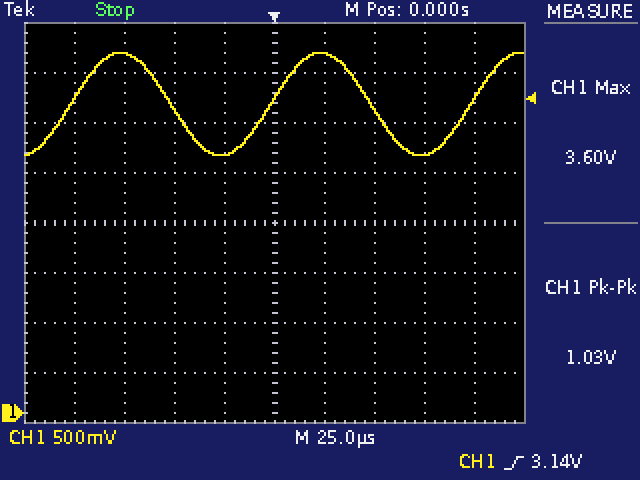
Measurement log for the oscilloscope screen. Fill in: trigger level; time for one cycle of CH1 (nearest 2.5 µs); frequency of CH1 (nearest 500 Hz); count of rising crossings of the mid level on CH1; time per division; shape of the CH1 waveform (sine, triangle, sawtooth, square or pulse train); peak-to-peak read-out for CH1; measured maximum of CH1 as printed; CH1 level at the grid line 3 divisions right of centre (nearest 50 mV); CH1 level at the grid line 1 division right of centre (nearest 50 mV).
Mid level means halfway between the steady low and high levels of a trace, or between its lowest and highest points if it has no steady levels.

3.14 V
100.0 µs
10.0 kHz
3
25 µs
sine
1.03 V
3.60 V
2.60 V
3.60 V
